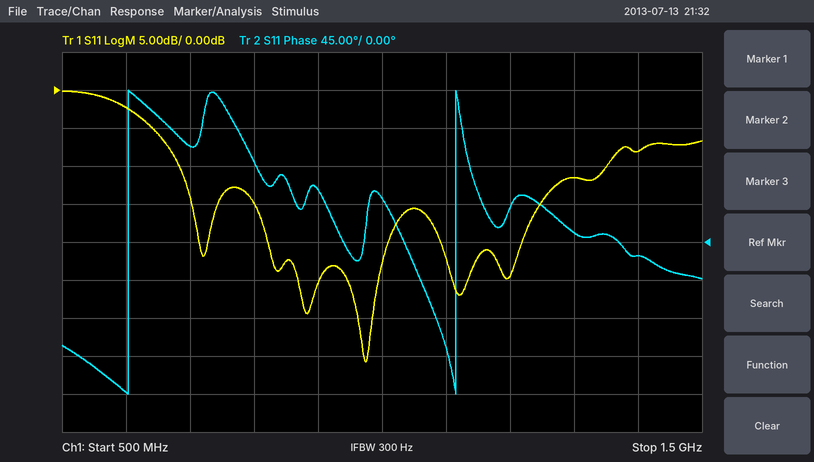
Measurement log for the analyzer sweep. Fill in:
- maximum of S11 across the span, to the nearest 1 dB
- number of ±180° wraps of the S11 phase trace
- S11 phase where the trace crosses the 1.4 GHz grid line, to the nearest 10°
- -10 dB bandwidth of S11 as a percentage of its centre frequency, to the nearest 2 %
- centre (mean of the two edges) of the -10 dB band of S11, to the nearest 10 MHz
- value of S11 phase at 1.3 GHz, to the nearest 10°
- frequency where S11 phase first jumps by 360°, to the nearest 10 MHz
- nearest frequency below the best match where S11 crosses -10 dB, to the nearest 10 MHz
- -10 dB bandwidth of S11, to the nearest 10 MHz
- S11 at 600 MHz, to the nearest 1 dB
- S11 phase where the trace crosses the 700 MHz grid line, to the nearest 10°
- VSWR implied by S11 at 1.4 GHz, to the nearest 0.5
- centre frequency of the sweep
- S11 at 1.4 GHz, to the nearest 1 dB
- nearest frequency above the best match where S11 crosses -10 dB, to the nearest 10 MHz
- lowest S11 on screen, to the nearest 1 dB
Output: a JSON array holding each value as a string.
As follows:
["0 dB", "2", "-20°", "66 %", "1.02 GHz", "10°", "600 MHz", "680 MHz", "670 MHz", "-2 dB", "110°", "2.5", "1 GHz", "-8 dB", "1.35 GHz", "-36 dB"]
